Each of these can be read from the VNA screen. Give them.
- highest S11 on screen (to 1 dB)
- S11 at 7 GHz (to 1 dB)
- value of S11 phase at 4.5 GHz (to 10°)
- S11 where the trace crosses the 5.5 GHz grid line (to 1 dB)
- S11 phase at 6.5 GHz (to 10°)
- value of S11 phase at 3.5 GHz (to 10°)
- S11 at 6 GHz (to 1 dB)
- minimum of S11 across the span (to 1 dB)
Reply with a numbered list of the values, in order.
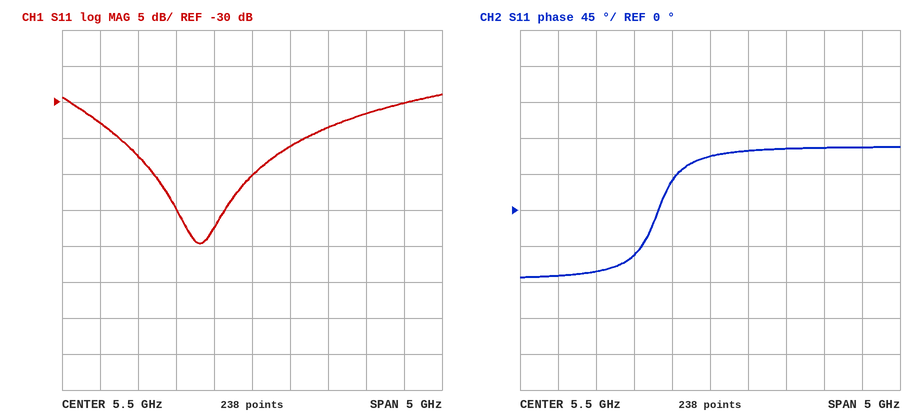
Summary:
1. -29 dB
2. -32 dB
3. -60°
4. -40 dB
5. 80°
6. -80°
7. -36 dB
8. -50 dB
